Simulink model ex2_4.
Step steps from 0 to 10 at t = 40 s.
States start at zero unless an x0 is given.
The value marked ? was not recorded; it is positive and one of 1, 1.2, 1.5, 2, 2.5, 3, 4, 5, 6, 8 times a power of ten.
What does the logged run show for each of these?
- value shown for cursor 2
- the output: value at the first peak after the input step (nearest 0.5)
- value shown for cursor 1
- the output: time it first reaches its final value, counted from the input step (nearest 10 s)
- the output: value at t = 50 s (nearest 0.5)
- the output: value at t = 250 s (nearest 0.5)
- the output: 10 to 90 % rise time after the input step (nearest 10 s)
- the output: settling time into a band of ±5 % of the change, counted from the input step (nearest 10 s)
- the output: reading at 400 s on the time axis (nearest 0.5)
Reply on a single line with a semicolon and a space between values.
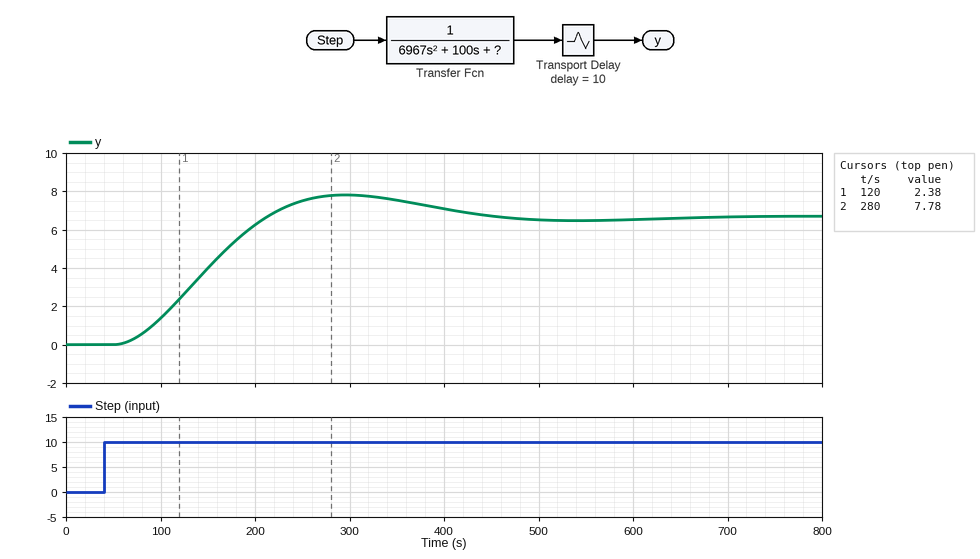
7.78; 8.0; 2.38; 170 s; 0.0; 7.5; 110 s; 370 s; 7.0
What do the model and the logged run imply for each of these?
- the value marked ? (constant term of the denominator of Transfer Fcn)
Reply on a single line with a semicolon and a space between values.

1.5
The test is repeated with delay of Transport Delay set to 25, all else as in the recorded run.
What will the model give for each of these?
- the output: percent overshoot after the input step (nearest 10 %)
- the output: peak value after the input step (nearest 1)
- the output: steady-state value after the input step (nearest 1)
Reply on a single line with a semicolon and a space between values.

20 %; 8; 7
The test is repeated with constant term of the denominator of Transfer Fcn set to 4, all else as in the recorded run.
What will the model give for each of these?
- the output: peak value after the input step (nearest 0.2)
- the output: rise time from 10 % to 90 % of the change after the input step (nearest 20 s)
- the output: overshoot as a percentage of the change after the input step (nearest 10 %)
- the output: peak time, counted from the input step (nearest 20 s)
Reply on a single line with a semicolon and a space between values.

3.4; 60 s; 40 %; 140 s
